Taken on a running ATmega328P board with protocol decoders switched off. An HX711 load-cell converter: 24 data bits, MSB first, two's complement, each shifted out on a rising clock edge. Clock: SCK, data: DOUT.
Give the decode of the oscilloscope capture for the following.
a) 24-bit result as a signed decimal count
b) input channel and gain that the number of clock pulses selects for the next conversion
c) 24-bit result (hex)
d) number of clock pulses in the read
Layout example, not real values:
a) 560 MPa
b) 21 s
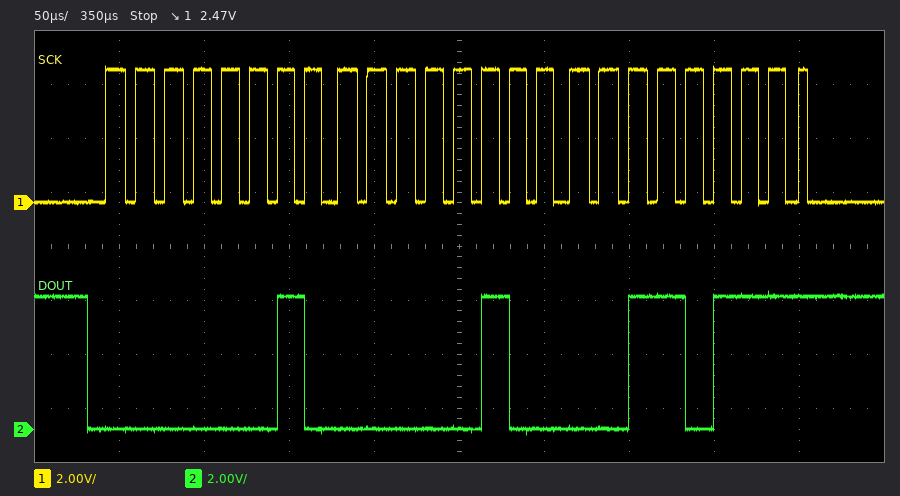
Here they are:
a) 132151
b) channel A, gain 128
c) 0x020437
d) 25
